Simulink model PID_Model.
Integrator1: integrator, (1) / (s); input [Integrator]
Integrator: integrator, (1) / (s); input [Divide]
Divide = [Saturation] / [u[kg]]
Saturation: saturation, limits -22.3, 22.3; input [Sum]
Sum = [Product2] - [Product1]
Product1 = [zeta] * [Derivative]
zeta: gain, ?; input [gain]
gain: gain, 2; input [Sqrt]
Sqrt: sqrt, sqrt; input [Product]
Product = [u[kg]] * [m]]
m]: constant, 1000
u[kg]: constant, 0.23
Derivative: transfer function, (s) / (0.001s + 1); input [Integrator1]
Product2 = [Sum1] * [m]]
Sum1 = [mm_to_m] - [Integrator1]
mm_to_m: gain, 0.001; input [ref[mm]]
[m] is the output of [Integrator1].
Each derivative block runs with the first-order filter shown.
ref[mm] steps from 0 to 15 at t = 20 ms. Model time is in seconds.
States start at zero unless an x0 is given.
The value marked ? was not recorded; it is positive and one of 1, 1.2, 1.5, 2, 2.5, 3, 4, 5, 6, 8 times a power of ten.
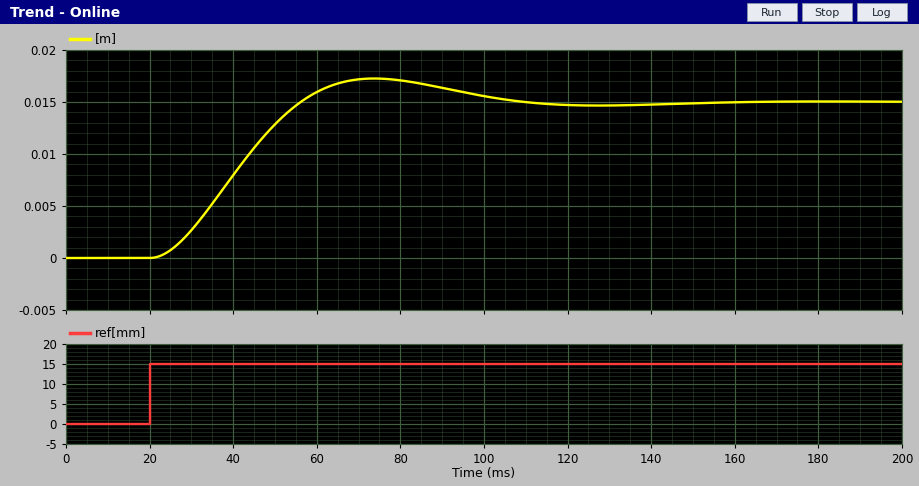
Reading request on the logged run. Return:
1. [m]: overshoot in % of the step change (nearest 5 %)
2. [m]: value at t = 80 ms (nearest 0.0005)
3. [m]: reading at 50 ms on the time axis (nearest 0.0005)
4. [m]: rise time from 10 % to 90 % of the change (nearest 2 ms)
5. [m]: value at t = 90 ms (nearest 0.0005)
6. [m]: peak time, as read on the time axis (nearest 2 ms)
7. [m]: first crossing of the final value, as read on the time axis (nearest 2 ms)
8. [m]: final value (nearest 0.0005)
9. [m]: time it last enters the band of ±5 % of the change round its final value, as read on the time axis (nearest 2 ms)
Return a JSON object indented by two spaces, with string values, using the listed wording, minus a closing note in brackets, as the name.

{
  "[m]: overshoot in % of the step change": "15 %",
  "[m]: value at t = 80 ms": "0.0170",
  "[m]: reading at 50 ms on the time axis": "0.0130",
  "[m]: rise time from 10 % to 90 % of the change": "24 ms",
  "[m]: value at t = 90 ms": "0.0165",
  "[m]: peak time, as read on the time axis": "74 ms",
  "[m]: first crossing of the final value, as read on the time axis": "56 ms",
  "[m]: final value": "0.0150",
  "[m]: time it last enters the band of ±5 % of the change round its final value, as read on the time axis": "98 ms"
}
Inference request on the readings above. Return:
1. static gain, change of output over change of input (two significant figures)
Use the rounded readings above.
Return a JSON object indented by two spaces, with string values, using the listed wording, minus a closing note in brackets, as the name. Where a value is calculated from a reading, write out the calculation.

{
  "static gain, change of output over change of input": "(0.015 - 0) / (15 - 0) = 0.0010"
}
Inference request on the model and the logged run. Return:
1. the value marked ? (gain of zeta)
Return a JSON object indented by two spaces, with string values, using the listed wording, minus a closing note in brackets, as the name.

{
  "the value marked ?": "0.5"
}
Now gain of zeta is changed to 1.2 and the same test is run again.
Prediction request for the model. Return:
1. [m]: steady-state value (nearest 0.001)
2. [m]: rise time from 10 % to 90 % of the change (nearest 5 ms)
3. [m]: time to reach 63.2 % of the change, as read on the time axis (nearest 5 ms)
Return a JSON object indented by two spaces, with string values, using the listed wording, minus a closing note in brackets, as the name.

{
  "[m]: steady-state value": "0.015",
  "[m]: rise time from 10 % to 90 % of the change": "70 ms",
  "[m]: time to reach 63.2 % of the change, as read on the time axis": "55 ms"
}
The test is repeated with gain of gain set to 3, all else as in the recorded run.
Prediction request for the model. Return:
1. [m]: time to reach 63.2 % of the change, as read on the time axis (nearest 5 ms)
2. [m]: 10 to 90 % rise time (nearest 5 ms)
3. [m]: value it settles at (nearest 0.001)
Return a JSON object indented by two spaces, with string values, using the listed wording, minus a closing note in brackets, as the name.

{
  "[m]: time to reach 63.2 % of the change, as read on the time axis": "45 ms",
  "[m]: 10 to 90 % rise time": "35 ms",
  "[m]: value it settles at": "0.015"
}
